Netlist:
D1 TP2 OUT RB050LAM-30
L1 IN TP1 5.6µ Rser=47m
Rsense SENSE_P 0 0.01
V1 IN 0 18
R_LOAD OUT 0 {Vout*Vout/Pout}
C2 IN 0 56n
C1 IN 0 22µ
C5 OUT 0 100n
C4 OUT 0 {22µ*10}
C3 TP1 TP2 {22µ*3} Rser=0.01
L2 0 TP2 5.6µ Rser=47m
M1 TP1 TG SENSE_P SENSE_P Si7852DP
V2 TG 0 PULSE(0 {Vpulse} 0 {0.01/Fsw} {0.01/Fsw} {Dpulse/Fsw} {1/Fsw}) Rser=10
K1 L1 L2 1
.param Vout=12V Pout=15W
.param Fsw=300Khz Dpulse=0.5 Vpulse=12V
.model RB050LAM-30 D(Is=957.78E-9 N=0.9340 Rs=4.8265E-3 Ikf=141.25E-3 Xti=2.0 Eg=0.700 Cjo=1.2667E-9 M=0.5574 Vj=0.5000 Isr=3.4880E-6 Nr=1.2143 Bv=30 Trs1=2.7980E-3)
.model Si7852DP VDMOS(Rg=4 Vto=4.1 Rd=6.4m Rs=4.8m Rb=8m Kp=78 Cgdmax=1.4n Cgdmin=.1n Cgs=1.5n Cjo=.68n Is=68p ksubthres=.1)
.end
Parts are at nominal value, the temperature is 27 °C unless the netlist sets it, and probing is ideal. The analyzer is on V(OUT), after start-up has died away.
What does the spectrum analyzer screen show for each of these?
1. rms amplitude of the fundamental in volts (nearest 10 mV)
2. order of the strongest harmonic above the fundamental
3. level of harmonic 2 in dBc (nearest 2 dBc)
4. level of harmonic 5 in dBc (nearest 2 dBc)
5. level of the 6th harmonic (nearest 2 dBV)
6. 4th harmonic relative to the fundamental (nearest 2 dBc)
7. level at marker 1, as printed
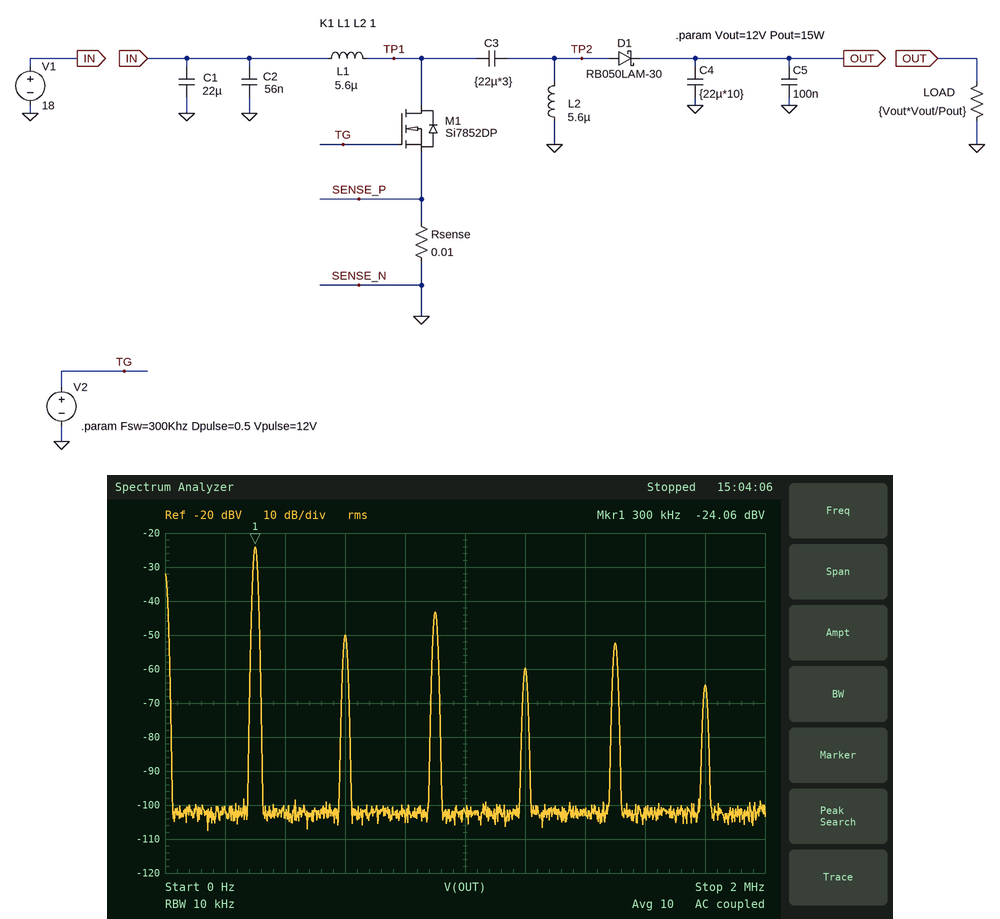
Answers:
60 mV
3
-26 dBc
-28 dBc
-64 dBV
-36 dBc
-24.06 dBV
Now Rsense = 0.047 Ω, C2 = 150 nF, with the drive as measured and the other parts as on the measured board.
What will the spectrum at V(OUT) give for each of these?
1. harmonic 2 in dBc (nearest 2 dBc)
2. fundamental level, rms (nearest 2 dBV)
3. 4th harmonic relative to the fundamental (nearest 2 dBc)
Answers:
-30 dBc
-28 dBV
-38 dBc
